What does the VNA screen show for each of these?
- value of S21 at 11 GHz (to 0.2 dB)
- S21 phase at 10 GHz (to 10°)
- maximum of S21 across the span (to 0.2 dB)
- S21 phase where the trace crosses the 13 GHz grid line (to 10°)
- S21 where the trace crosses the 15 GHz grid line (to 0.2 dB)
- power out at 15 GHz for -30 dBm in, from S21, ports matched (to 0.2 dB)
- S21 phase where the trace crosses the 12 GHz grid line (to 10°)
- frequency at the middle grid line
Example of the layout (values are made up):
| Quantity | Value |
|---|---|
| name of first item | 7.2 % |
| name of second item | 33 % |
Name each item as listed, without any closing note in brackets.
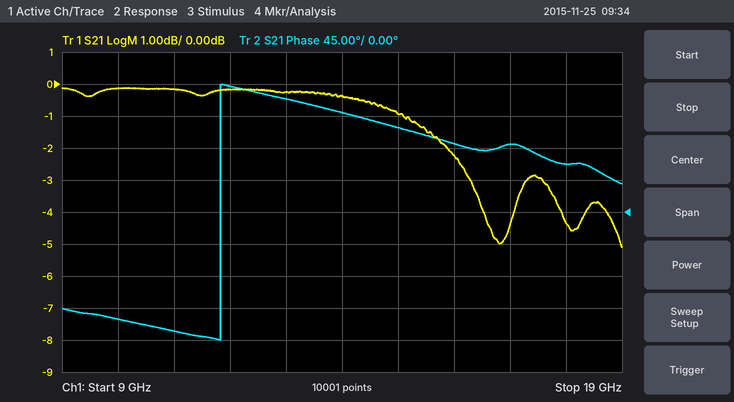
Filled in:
| Quantity | Value |
|---|---|
| value of S21 at 11 GHz | -0.2 dB |
| S21 phase at 10 GHz | -150° |
| maximum of S21 across the span | -0.2 dB |
| S21 phase where the trace crosses the 13 GHz grid line | 160° |
| S21 where the trace crosses the 15 GHz grid line | -1.0 dB |
| power out at 15 GHz for -30 dBm in, from S21, ports matched | -31.0 dBm |
| S21 phase where the trace crosses the 12 GHz grid line | 180° |
| frequency at the middle grid line | 14 GHz |
